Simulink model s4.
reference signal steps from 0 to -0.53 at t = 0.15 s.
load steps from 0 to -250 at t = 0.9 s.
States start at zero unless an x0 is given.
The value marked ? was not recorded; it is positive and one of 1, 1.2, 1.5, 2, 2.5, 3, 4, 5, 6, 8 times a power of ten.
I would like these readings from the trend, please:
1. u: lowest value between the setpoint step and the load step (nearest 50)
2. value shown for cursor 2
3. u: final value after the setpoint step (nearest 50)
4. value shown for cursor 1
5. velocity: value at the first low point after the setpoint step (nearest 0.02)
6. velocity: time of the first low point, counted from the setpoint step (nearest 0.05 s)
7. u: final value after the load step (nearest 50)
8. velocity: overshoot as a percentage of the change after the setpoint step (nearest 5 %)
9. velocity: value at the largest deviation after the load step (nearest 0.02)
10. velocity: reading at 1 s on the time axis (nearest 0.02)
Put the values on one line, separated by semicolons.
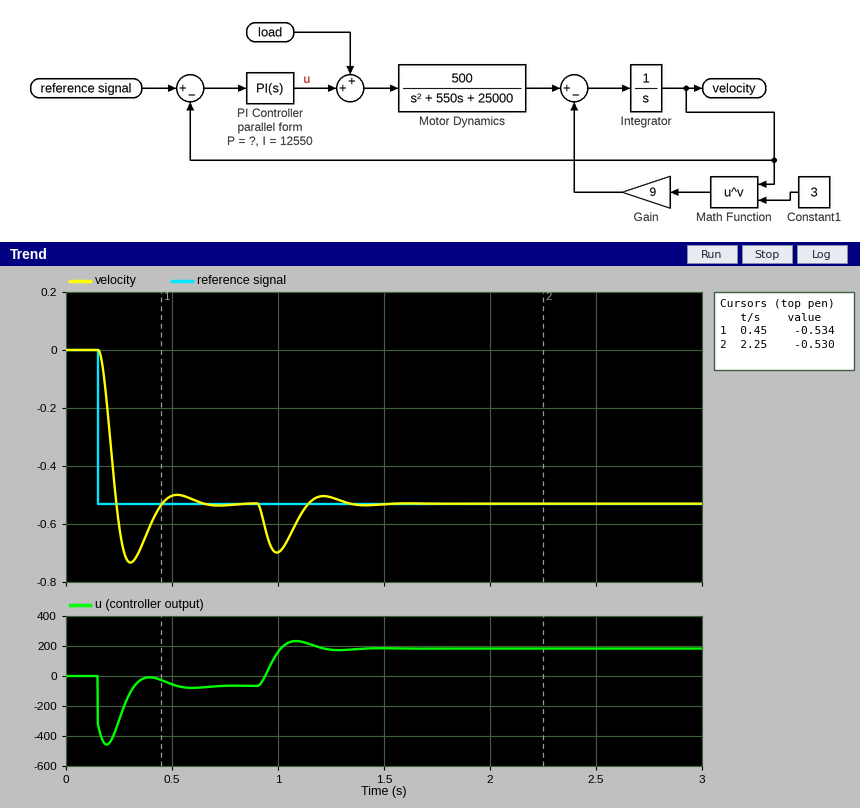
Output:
-450; -0.530; -50; -0.534; -0.74; 0.15 s; 200; 40 %; -0.70; -0.70
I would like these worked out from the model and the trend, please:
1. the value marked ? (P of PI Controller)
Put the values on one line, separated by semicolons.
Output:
600
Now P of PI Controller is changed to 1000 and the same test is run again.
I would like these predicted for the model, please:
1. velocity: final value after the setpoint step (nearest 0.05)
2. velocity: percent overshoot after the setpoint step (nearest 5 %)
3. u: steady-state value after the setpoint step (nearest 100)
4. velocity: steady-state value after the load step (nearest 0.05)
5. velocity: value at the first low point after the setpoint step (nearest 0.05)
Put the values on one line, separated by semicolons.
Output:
-0.55; 30 %; -100; -0.55; -0.70
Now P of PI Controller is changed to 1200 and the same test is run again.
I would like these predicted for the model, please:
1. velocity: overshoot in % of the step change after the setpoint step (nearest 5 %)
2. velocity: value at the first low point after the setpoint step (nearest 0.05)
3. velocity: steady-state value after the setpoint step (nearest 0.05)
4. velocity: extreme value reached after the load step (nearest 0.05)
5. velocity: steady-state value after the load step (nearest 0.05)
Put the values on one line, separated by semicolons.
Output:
25 %; -0.65; -0.55; -0.65; -0.55
